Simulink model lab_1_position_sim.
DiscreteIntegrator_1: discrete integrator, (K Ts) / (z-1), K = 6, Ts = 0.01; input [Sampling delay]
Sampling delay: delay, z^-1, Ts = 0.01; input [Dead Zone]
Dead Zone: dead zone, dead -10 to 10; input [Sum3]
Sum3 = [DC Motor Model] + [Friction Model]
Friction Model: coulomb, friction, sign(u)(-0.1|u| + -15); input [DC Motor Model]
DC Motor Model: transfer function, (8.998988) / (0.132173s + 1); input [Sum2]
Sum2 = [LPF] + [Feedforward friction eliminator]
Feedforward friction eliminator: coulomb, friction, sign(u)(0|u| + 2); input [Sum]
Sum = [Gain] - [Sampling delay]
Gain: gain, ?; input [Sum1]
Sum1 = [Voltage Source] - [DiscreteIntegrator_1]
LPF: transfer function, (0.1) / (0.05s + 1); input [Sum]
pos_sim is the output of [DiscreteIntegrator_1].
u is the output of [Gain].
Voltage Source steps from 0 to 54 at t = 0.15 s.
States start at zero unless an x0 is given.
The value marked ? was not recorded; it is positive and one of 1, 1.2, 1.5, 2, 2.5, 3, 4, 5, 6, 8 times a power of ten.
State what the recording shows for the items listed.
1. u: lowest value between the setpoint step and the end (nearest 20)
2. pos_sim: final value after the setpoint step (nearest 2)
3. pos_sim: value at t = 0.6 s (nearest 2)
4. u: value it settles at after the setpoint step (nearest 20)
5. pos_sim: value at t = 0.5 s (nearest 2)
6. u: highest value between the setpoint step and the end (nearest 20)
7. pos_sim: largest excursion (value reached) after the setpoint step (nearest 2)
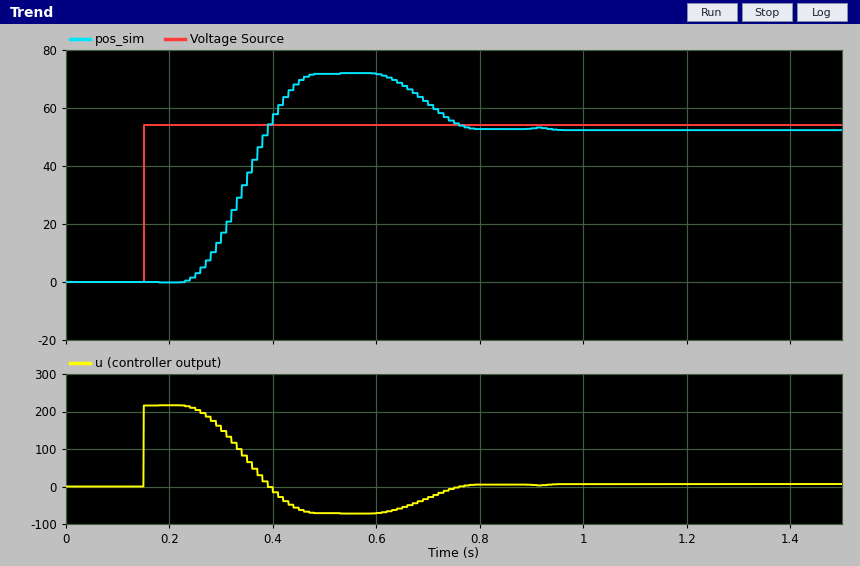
-80
52
72
0
72
220
72
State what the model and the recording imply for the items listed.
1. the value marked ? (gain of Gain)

4
